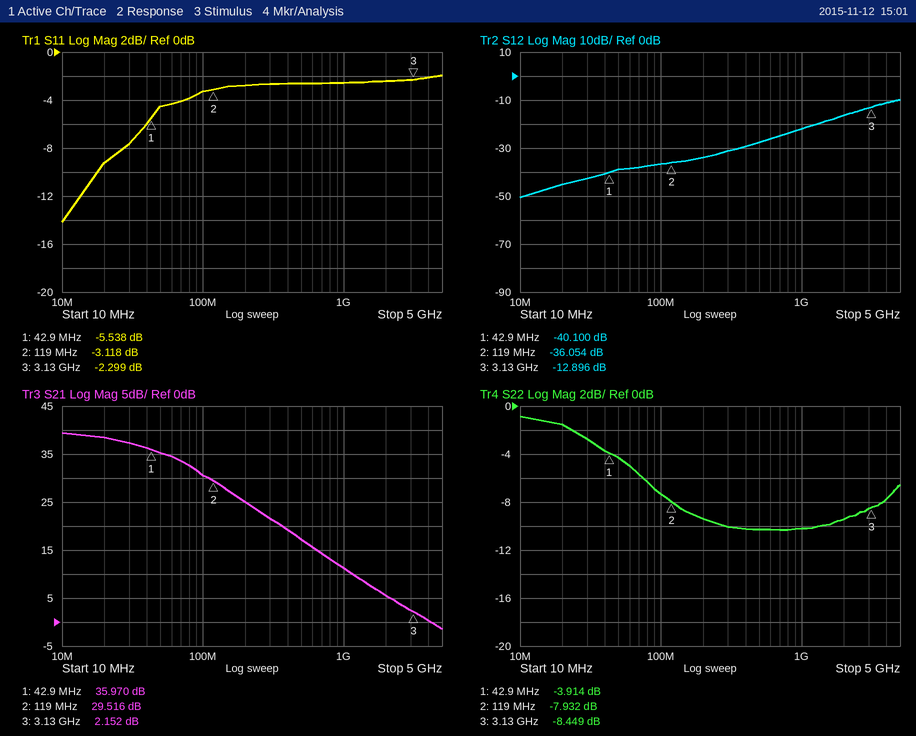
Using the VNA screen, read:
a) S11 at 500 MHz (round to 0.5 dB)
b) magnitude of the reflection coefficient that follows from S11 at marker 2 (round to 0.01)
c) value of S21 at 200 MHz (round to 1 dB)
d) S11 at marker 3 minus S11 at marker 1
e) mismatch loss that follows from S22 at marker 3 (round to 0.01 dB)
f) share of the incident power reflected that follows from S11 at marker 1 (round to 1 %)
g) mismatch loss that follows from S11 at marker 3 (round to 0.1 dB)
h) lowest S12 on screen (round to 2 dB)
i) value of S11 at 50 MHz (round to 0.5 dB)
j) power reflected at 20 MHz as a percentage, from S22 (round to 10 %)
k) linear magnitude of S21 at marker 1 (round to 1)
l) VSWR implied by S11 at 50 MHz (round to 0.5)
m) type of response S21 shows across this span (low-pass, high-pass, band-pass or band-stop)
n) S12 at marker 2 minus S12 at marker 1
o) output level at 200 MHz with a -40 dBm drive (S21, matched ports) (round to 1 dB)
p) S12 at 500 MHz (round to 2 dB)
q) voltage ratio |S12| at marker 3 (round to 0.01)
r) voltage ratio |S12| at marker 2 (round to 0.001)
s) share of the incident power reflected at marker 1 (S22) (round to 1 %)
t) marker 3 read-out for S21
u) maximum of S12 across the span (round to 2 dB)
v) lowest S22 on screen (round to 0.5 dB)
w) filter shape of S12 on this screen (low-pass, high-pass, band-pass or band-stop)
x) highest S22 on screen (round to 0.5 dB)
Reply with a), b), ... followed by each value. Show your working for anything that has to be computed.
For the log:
a) -2.5 dB
b) 10^(-3.118/20) ≈ 0.70
c) 25 dB
d) -2.299 − (-5.538) = 3.239 dB
e) −10 log10(1 − 10^(-8.449/10)) ≈ 0.67 dB
f) 10^(-5.538/10) ≈ 28 %
g) −10 log10(1 − 10^(-2.299/10)) ≈ 3.9 dB
h) -50 dB
i) -4.5 dB
j) 10^(-1.5/10) ≈ 70.8 %, so 70 % to the nearest 10 %
k) 10^(35.97/20) ≈ 63
l) |Γ| = 10^(-4.5/20) = 0.5957; VSWR = (1 + 0.5957)/(1 − 0.5957) ≈ 4.0
m) low-pass
n) -36.054 − (-40.1) = 4.046 dB
o) -40 dBm + (25 dB) = -15 dBm
p) -28 dB
q) 10^(-12.896/20) ≈ 0.23
r) 10^(-36.054/20) ≈ 0.016
s) 10^(-3.914/10) ≈ 41 %
t) 2.152 dB
u) -10 dB
v) -10.5 dB
w) high-pass
x) -1.0 dB
